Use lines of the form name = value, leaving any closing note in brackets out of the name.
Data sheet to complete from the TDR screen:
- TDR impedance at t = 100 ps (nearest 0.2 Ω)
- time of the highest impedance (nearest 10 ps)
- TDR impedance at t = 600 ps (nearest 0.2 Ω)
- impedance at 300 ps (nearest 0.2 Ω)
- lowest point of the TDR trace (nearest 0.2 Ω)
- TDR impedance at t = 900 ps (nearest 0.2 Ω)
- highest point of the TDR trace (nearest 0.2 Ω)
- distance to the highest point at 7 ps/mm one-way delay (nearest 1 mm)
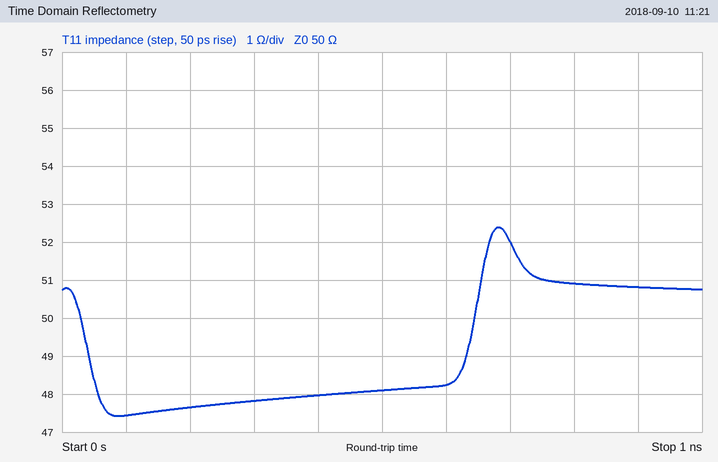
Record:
TDR impedance at t = 100 ps = 47.4 Ω
time of the highest impedance = 680 ps
TDR impedance at t = 600 ps = 48.2 Ω
impedance at 300 ps = 47.8 Ω
lowest point of the TDR trace = 47.4 Ω
TDR impedance at t = 900 ps = 50.8 Ω
highest point of the TDR trace = 52.4 Ω
distance to the highest point at 7 ps/mm one-way delay = 49 mm
